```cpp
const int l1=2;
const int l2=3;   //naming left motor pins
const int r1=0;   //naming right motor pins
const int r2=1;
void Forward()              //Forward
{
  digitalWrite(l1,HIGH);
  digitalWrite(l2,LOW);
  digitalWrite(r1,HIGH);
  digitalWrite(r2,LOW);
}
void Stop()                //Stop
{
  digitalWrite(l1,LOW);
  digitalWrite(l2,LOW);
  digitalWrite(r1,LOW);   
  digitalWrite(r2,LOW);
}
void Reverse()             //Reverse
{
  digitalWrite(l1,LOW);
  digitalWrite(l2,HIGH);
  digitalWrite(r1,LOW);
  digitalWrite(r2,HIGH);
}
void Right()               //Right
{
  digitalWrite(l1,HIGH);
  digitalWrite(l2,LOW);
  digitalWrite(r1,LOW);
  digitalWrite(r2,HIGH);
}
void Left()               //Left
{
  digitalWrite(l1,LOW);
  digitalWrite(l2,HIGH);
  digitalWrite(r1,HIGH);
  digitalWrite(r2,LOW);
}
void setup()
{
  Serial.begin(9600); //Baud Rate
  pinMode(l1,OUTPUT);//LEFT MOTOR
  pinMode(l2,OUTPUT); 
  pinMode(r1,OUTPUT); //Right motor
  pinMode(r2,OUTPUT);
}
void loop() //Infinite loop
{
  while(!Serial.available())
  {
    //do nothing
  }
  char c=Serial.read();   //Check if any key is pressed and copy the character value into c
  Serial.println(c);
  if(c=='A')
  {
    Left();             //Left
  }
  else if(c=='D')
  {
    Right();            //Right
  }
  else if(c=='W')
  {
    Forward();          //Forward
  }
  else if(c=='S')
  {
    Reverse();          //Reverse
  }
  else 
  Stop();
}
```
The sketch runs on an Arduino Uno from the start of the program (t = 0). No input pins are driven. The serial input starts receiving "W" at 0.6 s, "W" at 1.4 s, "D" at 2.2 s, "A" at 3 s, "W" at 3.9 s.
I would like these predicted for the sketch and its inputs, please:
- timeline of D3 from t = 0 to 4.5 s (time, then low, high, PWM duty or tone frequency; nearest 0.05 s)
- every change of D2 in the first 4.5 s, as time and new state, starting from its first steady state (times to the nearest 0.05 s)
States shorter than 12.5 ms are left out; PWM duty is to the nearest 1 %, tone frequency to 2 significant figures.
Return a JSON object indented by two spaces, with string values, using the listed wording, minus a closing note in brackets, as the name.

{
  "timeline of D3 from t = 0 to 4.5 s": "0 s low; 3 s high; 3.9 s low",
  "every change of D2 in the first 4.5 s, as time and new state, starting from its first steady state": "0 s low; 0.6 s high; 3 s low; 3.9 s high"
}
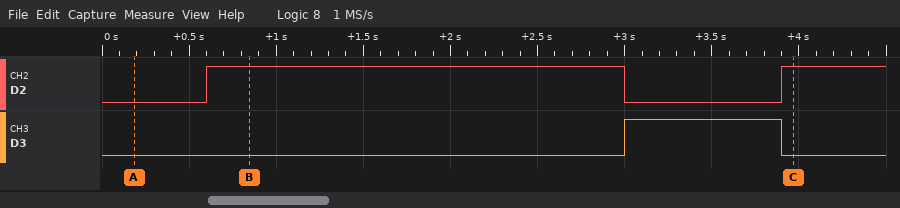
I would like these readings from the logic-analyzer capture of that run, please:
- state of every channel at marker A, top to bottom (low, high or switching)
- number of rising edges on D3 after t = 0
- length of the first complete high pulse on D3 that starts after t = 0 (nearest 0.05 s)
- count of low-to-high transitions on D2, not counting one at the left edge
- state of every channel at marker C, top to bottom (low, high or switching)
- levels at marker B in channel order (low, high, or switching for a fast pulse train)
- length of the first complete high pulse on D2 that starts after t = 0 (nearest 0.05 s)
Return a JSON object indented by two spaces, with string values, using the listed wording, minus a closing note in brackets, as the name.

{
  "state of every channel at marker A, top to bottom": "D2 low, D3 low",
  "number of rising edges on D3 after t = 0": "1",
  "length of the first complete high pulse on D3 that starts after t = 0": "0.90 s",
  "count of low-to-high transitions on D2, not counting one at the left edge": "2",
  "state of every channel at marker C, top to bottom": "D2 high, D3 low",
  "levels at marker B in channel order": "D2 high, D3 low",
  "length of the first complete high pulse on D2 that starts after t = 0": "2.40 s"
}
